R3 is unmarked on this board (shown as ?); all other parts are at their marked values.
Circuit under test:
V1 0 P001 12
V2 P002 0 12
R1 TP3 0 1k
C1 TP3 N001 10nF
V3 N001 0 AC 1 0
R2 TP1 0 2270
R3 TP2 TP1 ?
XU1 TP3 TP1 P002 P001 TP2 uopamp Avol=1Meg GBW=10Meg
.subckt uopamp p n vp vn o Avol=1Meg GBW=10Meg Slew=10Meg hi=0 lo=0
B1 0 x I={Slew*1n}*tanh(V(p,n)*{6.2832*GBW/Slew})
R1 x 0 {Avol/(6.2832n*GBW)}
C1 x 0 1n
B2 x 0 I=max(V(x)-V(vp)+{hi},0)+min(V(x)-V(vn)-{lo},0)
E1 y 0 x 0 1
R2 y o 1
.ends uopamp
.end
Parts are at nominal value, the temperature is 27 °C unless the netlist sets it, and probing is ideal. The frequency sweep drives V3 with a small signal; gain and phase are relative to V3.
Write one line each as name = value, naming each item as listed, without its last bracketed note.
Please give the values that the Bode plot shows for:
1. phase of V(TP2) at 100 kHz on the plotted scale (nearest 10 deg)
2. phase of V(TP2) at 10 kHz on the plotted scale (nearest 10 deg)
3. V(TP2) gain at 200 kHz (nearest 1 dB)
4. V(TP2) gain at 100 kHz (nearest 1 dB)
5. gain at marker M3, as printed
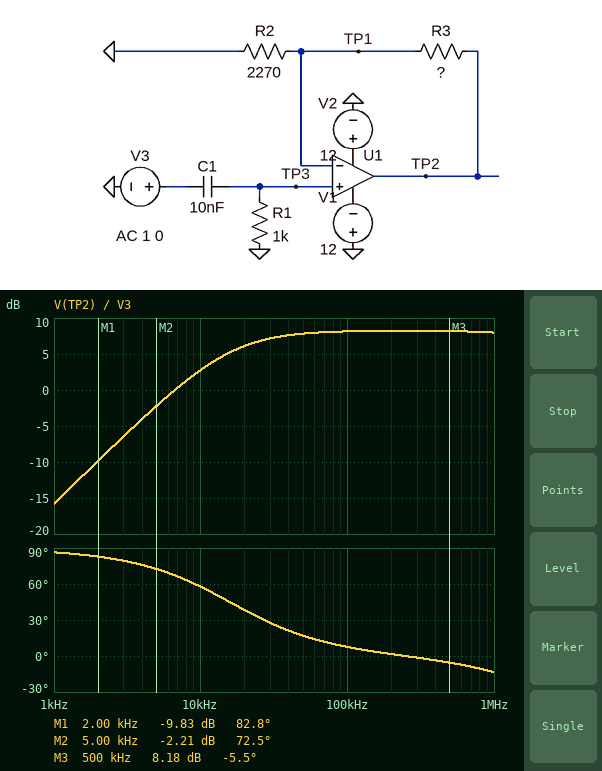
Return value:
phase of V(TP2) at 100 kHz on the plotted scale = 10 deg
phase of V(TP2) at 10 kHz on the plotted scale = 60 deg
V(TP2) gain at 200 kHz = 8 dB
V(TP2) gain at 100 kHz = 8 dB
gain at marker M3, as printed = 8.18 dB
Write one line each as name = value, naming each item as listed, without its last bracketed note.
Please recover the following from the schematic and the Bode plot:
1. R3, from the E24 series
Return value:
R3, from the E24 series = 3.6 kΩ
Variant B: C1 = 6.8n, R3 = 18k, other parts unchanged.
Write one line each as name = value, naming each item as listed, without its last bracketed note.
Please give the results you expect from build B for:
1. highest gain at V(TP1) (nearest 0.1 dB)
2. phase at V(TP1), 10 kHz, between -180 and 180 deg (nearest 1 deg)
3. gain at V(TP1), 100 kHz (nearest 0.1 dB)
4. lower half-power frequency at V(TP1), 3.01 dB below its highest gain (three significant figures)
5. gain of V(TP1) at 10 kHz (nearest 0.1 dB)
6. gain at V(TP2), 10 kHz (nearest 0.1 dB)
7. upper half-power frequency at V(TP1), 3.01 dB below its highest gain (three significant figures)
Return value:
highest gain at V(TP1) = -0.2 dB
phase at V(TP1), 10 kHz, between -180 and 180 deg = 66 deg
gain at V(TP1), 100 kHz = -0.3 dB
lower half-power frequency at V(TP1), 3.01 dB below its highest gain = 22.5 kHz
gain of V(TP1) at 10 kHz = -8.1 dB
gain at V(TP2), 10 kHz = 10.9 dB
upper half-power frequency at V(TP1), 3.01 dB below its highest gain = 1.17 MHz
